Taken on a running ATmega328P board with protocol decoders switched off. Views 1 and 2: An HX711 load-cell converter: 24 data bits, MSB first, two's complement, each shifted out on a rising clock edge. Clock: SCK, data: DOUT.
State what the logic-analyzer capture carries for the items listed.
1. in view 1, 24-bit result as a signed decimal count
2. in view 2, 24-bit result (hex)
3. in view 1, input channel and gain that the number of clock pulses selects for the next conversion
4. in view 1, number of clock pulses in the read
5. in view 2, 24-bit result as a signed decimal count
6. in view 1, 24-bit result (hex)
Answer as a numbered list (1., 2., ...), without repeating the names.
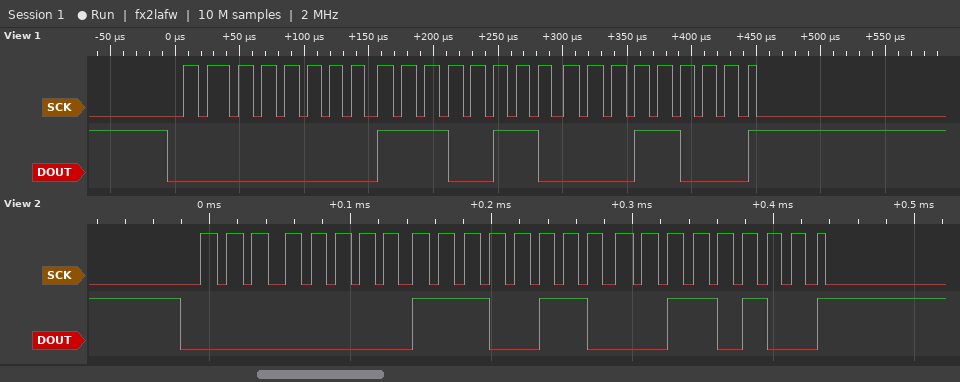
1. 58904
2. 0x00E634
3. channel A, gain 128
4. 25
5. 58932
6. 0x00E618
